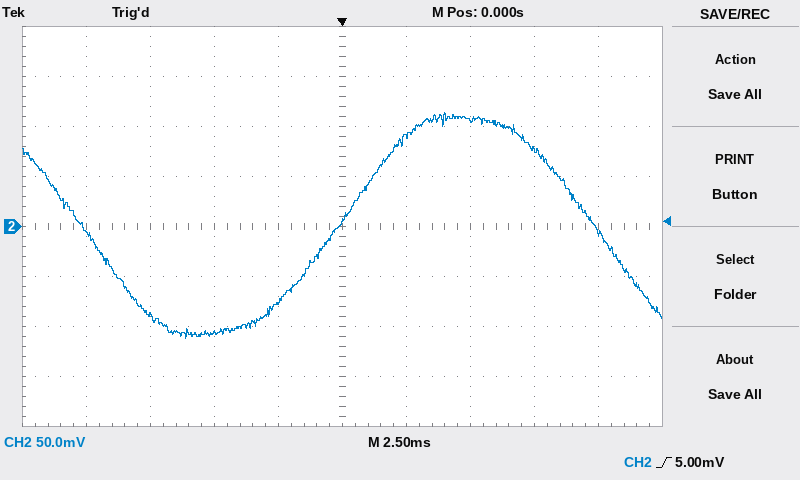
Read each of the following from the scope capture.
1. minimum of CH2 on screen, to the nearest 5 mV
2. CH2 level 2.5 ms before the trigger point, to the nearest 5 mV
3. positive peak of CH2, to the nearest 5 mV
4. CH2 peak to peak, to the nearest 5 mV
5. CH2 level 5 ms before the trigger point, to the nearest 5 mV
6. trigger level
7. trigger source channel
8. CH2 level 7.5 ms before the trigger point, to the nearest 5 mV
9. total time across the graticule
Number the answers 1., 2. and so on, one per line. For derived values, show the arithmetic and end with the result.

1. -110 mV
2. -75 mV
3. 115 mV
4. 115 mV − (-110 mV) = 225 mV
5. -105 mV
6. 5.00 mV
7. CH2
8. -90 mV
9. 25 ms
